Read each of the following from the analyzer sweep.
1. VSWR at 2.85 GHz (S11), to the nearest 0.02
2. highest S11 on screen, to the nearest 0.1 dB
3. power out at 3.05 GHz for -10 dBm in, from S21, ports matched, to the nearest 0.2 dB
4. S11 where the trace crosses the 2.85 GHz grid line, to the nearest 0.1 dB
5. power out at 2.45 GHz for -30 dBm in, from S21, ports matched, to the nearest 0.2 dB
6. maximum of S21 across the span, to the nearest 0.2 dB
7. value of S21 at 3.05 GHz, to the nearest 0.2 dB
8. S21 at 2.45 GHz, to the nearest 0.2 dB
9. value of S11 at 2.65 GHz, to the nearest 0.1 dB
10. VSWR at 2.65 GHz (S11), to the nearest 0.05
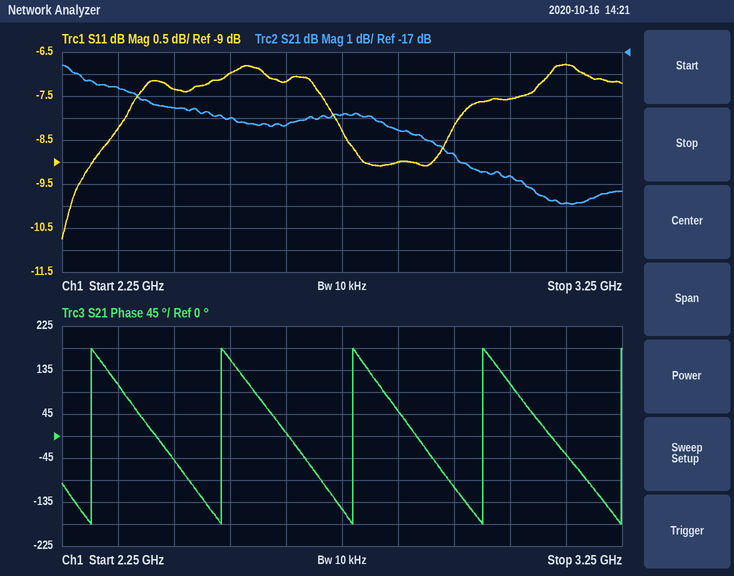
2.10
-6.8 dB
-32.6 dBm
-9.0 dB
-49.6 dBm
-17.6 dB
-22.6 dB
-19.6 dB
-7.2 dB
2.55
